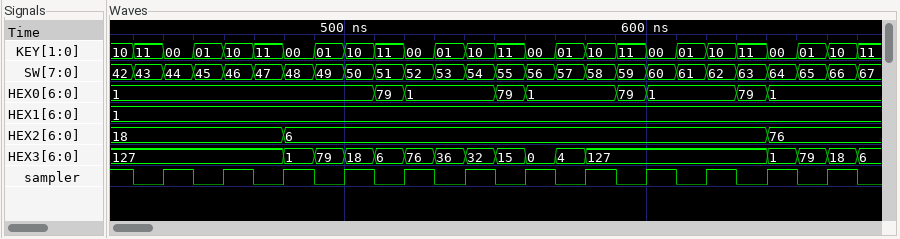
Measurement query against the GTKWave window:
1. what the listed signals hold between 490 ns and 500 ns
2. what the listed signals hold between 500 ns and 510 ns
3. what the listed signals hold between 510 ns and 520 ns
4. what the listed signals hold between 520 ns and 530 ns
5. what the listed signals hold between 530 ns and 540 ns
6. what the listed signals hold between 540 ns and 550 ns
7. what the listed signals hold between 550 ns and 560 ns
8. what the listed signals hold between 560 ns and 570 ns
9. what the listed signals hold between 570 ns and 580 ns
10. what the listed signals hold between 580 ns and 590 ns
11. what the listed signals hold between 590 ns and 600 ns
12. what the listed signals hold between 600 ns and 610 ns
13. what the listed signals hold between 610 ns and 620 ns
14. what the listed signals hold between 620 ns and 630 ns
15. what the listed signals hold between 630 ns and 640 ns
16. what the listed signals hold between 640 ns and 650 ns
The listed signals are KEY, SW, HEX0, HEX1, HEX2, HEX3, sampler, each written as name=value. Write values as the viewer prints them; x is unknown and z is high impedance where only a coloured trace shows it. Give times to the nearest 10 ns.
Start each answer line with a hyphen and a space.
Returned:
- KEY=01, SW=49, HEX0=1, HEX1=1, HEX2=6, HEX3=79, sampler=0
- KEY=10, SW=50, HEX0=1, HEX1=1, HEX2=6, HEX3=18, sampler=1
- KEY=11, SW=51, HEX0=79, HEX1=1, HEX2=6, HEX3=6, sampler=0
- KEY=00, SW=52, HEX0=1, HEX1=1, HEX2=6, HEX3=76, sampler=1
- KEY=01, SW=53, HEX0=1, HEX1=1, HEX2=6, HEX3=36, sampler=0
- KEY=10, SW=54, HEX0=1, HEX1=1, HEX2=6, HEX3=32, sampler=1
- KEY=11, SW=55, HEX0=79, HEX1=1, HEX2=6, HEX3=15, sampler=0
- KEY=00, SW=56, HEX0=1, HEX1=1, HEX2=6, HEX3=0, sampler=1
- KEY=01, SW=57, HEX0=1, HEX1=1, HEX2=6, HEX3=4, sampler=0
- KEY=10, SW=58, HEX0=1, HEX1=1, HEX2=6, HEX3=127, sampler=1
- KEY=11, SW=59, HEX0=79, HEX1=1, HEX2=6, HEX3=127, sampler=0
- KEY=00, SW=60, HEX0=1, HEX1=1, HEX2=6, HEX3=127, sampler=1
- KEY=01, SW=61, HEX0=1, HEX1=1, HEX2=6, HEX3=127, sampler=0
- KEY=10, SW=62, HEX0=1, HEX1=1, HEX2=6, HEX3=127, sampler=1
- KEY=11, SW=63, HEX0=79, HEX1=1, HEX2=6, HEX3=127, sampler=0
- KEY=00, SW=64, HEX0=1, HEX1=1, HEX2=76, HEX3=1, sampler=1
